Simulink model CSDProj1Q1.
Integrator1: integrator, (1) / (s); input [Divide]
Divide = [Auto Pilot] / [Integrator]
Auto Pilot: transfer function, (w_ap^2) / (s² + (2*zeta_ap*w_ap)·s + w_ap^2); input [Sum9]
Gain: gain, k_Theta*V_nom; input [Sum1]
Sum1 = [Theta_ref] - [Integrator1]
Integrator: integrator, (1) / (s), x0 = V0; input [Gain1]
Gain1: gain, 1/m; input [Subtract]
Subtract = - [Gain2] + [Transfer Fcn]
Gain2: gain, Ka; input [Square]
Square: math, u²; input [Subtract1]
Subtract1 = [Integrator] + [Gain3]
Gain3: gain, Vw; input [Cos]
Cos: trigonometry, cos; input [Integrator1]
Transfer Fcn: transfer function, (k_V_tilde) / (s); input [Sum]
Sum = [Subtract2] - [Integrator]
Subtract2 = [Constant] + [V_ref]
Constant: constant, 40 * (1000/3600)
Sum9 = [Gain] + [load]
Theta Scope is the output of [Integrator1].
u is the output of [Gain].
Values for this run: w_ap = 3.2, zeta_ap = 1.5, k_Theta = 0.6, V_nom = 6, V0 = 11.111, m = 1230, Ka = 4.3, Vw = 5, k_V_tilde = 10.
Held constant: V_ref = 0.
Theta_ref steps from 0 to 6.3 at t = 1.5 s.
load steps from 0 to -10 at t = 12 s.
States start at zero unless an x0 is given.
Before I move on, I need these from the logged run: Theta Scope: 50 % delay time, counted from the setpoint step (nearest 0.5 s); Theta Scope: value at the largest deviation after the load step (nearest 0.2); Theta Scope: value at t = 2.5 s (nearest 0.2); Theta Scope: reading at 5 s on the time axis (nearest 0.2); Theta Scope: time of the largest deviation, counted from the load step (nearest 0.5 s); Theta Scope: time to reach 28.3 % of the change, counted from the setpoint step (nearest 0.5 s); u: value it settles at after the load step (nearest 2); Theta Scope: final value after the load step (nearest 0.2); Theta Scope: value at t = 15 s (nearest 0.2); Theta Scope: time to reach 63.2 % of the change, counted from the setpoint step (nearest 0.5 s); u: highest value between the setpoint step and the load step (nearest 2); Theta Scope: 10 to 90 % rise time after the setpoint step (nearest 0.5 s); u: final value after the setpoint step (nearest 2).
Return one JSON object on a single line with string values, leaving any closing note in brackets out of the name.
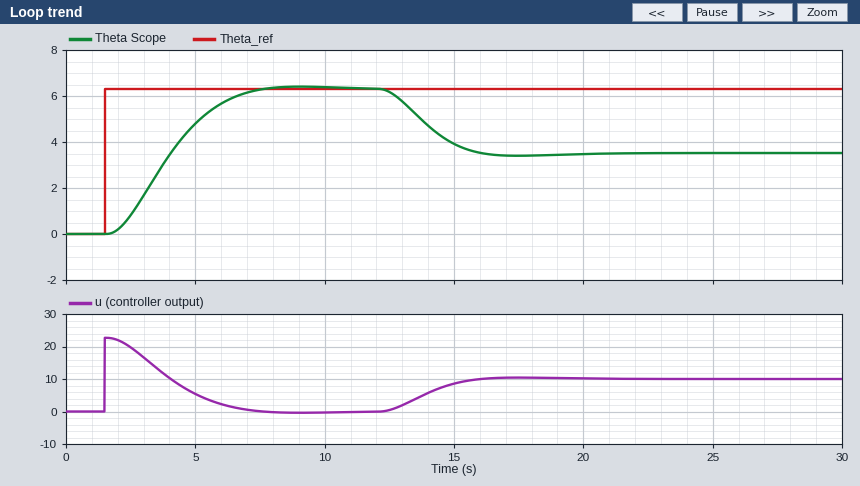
{"Theta Scope: 50 % delay time, counted from the setpoint step": "2.5 s", "Theta Scope: value at the largest deviation after the load step": "3.4", "Theta Scope: value at t = 2.5 s": "0.8", "Theta Scope: reading at 5 s on the time axis": "4.8", "Theta Scope: time of the largest deviation, counted from the load step": "5.5 s", "Theta Scope: time to reach 28.3 % of the change, counted from the setpoint step": "1.5 s", "u: value it settles at after the load step": "10", "Theta Scope: final value after the load step": "3.6", "Theta Scope: value at t = 15 s": "4.0", "Theta Scope: time to reach 63.2 % of the change, counted from the setpoint step": "3.0 s", "u: highest value between the setpoint step and the load step": "22", "Theta Scope: 10 to 90 % rise time after the setpoint step": "3.5 s", "u: final value after the setpoint step": "0"}
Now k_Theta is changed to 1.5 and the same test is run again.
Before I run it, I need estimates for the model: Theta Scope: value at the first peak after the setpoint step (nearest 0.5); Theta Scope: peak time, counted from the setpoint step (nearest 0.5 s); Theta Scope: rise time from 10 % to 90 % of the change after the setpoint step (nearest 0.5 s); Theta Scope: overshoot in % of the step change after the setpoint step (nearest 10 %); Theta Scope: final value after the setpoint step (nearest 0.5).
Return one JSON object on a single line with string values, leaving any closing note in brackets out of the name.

{"Theta Scope: value at the first peak after the setpoint step": "7.5", "Theta Scope: peak time, counted from the setpoint step": "3.5 s", "Theta Scope: rise time from 10 % to 90 % of the change after the setpoint step": "1.5 s", "Theta Scope: overshoot in % of the step change after the setpoint step": "20 %", "Theta Scope: final value after the setpoint step": "6.5"}
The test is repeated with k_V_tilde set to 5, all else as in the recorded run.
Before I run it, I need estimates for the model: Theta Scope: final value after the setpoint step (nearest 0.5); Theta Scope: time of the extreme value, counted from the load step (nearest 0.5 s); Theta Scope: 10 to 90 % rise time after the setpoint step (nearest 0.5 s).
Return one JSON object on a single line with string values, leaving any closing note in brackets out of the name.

{"Theta Scope: final value after the setpoint step": "6.5", "Theta Scope: time of the extreme value, counted from the load step": "5.0 s", "Theta Scope: 10 to 90 % rise time after the setpoint step": "3.5 s"}
